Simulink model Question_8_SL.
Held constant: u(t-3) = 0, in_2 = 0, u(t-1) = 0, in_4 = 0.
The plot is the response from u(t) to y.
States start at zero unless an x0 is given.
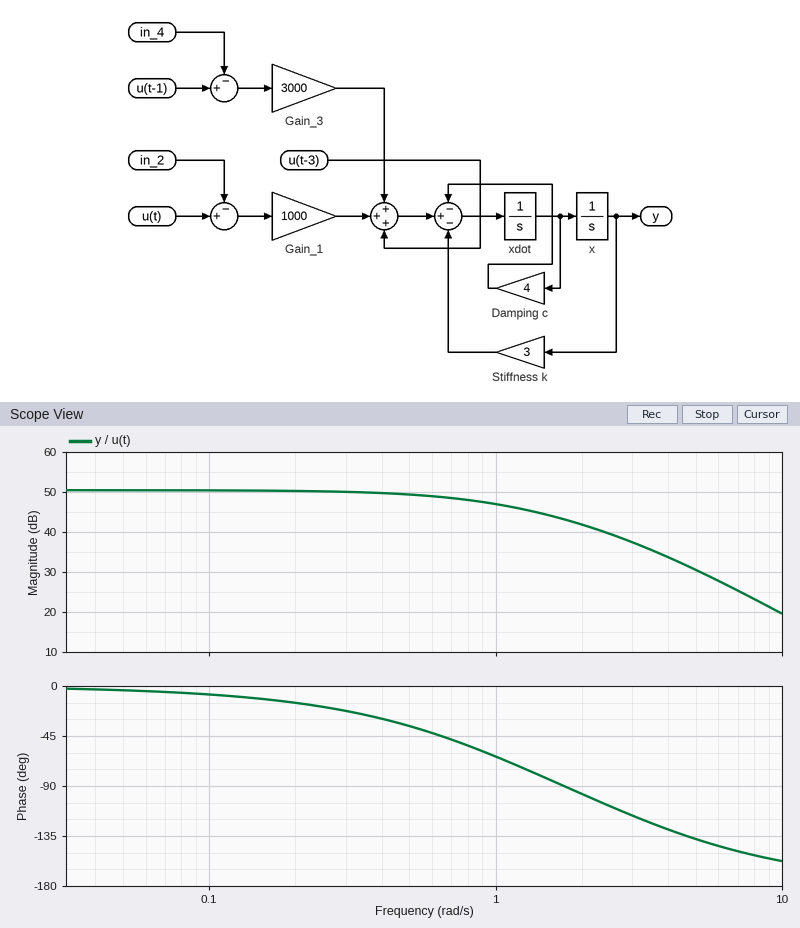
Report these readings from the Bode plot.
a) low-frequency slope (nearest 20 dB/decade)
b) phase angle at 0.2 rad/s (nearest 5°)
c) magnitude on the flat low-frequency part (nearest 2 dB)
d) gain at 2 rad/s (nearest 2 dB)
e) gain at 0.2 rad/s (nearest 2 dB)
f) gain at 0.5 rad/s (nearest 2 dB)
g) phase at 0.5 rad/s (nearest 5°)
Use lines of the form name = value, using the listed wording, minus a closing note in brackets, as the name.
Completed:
low-frequency slope = 0 dB/decade
phase angle at 0.2 rad/s = -15°
magnitude on the flat low-frequency part = 50 dB
gain at 2 rad/s = 42 dB
gain at 0.2 rad/s = 50 dB
gain at 0.5 rad/s = 50 dB
phase at 0.5 rad/s = -35°
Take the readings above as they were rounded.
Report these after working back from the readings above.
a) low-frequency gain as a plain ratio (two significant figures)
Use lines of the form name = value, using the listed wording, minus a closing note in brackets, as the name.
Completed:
low-frequency gain as a plain ratio = 320
